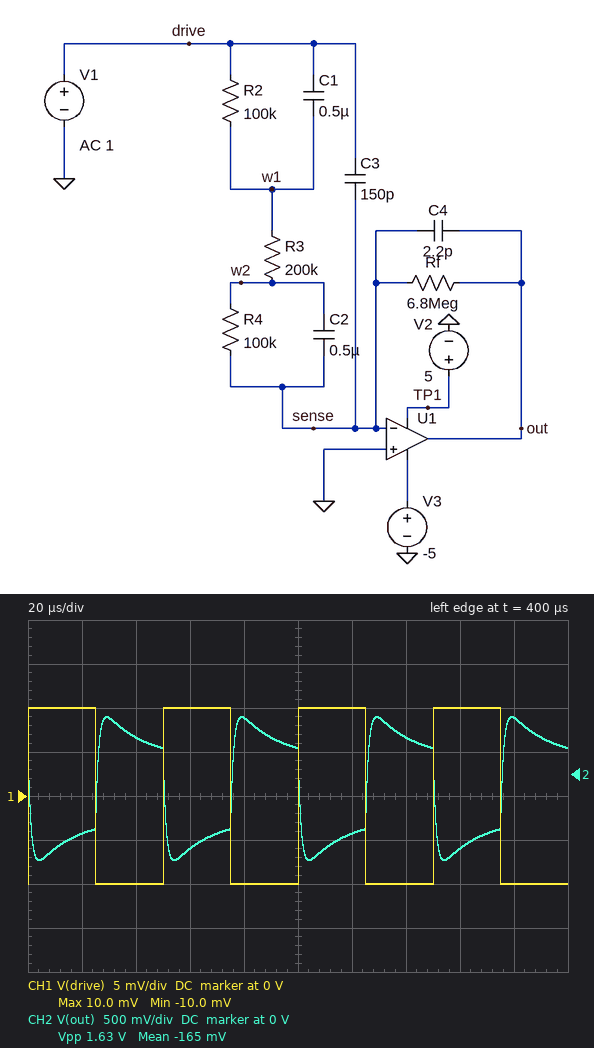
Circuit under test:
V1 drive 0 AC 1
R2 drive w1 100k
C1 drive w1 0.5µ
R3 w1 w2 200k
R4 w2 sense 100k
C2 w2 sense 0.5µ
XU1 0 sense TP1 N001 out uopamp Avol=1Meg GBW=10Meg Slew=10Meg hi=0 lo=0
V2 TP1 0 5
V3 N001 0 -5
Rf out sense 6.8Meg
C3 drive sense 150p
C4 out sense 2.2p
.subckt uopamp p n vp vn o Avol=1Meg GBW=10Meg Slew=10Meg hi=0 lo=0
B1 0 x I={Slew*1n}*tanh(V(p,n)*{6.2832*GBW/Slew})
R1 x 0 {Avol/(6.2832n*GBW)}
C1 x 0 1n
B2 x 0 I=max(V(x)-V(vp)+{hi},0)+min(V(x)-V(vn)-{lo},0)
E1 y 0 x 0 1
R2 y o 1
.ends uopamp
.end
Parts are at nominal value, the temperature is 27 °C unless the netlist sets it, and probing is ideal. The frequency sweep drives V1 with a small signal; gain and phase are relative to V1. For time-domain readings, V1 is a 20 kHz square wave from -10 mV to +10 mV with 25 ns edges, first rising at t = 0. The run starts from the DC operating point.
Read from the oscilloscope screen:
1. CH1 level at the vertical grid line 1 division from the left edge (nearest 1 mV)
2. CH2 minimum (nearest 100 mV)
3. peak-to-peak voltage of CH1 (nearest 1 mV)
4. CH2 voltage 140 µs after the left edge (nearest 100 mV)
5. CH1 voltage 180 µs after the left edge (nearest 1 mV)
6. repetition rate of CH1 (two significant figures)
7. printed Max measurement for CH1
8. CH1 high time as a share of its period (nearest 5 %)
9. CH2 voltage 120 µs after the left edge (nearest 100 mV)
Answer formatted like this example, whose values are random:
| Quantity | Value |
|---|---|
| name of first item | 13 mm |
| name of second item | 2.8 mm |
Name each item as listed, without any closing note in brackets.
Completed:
| Quantity | Value |
|---|---|
| CH1 level at the vertical grid line 1 division from the left edge | 10 mV |
| CH2 minimum | -1.0 V |
| peak-to-peak voltage of CH1 | 20 mV |
| CH2 voltage 140 µs after the left edge | 400 mV |
| CH1 voltage 180 µs after the left edge | -10 mV |
| repetition rate of CH1 | 20 kHz |
| printed Max measurement for CH1 | 10.0 mV |
| CH1 high time as a share of its period | 50 % |
| CH2 voltage 120 µs after the left edge | -700 mV |
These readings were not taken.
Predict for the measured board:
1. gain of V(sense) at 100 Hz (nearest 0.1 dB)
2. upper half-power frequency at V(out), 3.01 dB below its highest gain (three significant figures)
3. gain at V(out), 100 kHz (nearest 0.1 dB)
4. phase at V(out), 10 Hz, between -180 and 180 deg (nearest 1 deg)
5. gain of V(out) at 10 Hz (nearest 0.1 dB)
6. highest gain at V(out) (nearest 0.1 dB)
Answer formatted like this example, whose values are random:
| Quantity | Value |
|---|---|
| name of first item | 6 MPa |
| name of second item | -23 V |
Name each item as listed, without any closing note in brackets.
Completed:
| Quantity | Value |
|---|---|
| gain of V(sense) at 100 Hz | -69.3 dB |
| upper half-power frequency at V(out), 3.01 dB below its highest gain | 157 kHz |
| gain at V(out), 100 kHz | 35.2 dB |
| phase at V(out), 10 Hz, between -180 and 180 deg | -165 deg |
| gain of V(out) at 10 Hz | 29.6 dB |
| highest gain at V(out) | 36.4 dB |
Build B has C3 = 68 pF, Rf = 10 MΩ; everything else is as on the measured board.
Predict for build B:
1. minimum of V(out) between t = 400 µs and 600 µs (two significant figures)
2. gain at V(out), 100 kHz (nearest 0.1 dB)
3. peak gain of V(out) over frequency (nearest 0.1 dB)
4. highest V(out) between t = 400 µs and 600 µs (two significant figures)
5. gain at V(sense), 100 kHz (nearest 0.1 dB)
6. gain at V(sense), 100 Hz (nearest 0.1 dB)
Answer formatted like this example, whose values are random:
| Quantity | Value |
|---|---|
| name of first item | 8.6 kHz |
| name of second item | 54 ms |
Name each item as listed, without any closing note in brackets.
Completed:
| Quantity | Value |
|---|---|
| minimum of V(out) between t = 400 µs and 600 µs | -650 mV |
| gain at V(out), 100 kHz | 29.3 dB |
| peak gain of V(out) over frequency | 34.0 dB |
| highest V(out) between t = 400 µs and 600 µs | 160 mV |
| gain at V(sense), 100 kHz | -10.7 dB |
| gain at V(sense), 100 Hz | -66.0 dB |
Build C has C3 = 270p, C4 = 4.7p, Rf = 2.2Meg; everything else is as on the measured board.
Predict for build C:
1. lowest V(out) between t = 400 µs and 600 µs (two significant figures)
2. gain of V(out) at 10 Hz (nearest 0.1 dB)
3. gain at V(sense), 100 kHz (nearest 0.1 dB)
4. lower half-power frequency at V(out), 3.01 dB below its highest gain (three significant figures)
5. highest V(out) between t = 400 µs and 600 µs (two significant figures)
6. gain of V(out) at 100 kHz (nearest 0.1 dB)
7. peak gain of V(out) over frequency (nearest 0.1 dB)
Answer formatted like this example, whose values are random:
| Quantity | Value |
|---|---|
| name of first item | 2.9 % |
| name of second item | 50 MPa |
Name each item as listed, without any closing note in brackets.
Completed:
| Quantity | Value |
|---|---|
| lowest V(out) between t = 400 µs and 600 µs | -880 mV |
| gain of V(out) at 10 Hz | 19.8 dB |
| gain at V(sense), 100 kHz | -5.7 dB |
| lower half-power frequency at V(out), 3.01 dB below its highest gain | 13.5 kHz |
| highest V(out) between t = 400 µs and 600 µs | 770 mV |
| gain of V(out) at 100 kHz | 34.3 dB |
| peak gain of V(out) over frequency | 35.0 dB |
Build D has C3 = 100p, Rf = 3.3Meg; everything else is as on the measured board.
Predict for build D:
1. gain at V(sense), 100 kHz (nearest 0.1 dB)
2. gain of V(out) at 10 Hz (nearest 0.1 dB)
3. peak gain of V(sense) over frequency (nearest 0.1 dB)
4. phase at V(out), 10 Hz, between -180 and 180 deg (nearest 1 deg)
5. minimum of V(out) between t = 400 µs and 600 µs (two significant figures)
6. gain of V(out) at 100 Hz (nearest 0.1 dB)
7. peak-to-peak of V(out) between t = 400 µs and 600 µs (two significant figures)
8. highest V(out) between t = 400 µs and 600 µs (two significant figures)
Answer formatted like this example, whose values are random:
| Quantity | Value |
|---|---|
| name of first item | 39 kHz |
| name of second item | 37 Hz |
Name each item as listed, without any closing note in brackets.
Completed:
| Quantity | Value |
|---|---|
| gain at V(sense), 100 kHz | -7.4 dB |
| gain of V(out) at 10 Hz | 23.3 dB |
| peak gain of V(sense) over frequency | -0.2 dB |
| phase at V(out), 10 Hz, between -180 and 180 deg | -165 deg |
| minimum of V(out) between t = 400 µs and 600 µs | -700 mV |
| gain of V(out) at 100 Hz | 24.3 dB |
| peak-to-peak of V(out) between t = 400 µs and 600 µs | 1.2 V |
| highest V(out) between t = 400 µs and 600 µs | 540 mV |
